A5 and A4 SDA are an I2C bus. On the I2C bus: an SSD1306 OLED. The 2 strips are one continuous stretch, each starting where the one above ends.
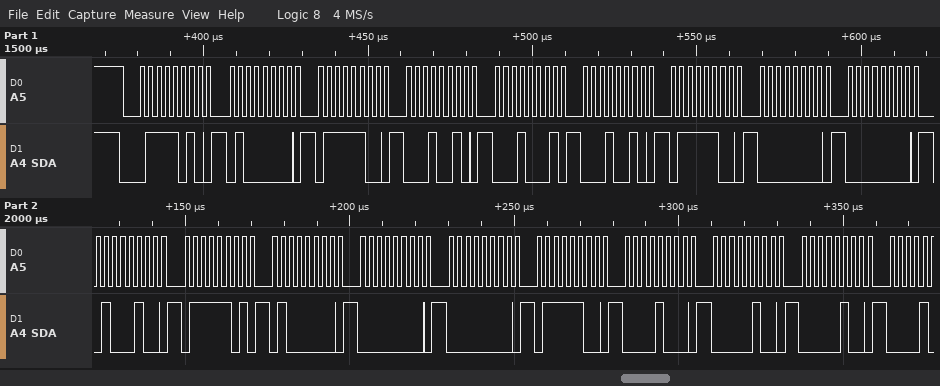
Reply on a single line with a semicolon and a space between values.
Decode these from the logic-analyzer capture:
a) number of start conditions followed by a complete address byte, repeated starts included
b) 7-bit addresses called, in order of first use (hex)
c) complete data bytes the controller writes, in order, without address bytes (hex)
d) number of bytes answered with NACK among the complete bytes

1; 0x3D; 40 7C 12 11 12 7C 00 00 44 7D 40 00 00 7C 08 04 04; 0
